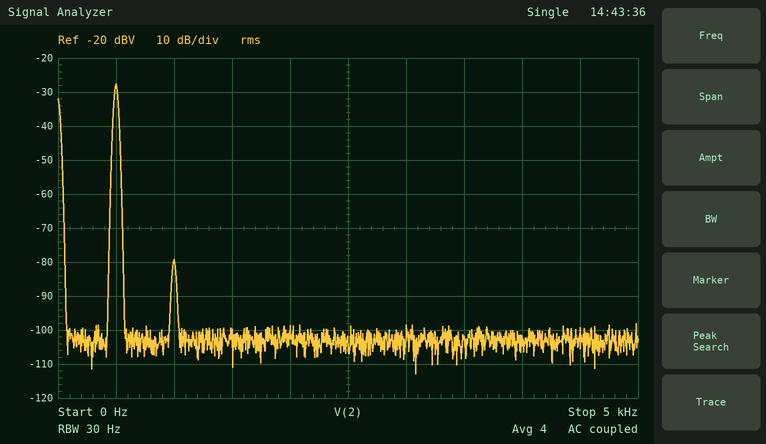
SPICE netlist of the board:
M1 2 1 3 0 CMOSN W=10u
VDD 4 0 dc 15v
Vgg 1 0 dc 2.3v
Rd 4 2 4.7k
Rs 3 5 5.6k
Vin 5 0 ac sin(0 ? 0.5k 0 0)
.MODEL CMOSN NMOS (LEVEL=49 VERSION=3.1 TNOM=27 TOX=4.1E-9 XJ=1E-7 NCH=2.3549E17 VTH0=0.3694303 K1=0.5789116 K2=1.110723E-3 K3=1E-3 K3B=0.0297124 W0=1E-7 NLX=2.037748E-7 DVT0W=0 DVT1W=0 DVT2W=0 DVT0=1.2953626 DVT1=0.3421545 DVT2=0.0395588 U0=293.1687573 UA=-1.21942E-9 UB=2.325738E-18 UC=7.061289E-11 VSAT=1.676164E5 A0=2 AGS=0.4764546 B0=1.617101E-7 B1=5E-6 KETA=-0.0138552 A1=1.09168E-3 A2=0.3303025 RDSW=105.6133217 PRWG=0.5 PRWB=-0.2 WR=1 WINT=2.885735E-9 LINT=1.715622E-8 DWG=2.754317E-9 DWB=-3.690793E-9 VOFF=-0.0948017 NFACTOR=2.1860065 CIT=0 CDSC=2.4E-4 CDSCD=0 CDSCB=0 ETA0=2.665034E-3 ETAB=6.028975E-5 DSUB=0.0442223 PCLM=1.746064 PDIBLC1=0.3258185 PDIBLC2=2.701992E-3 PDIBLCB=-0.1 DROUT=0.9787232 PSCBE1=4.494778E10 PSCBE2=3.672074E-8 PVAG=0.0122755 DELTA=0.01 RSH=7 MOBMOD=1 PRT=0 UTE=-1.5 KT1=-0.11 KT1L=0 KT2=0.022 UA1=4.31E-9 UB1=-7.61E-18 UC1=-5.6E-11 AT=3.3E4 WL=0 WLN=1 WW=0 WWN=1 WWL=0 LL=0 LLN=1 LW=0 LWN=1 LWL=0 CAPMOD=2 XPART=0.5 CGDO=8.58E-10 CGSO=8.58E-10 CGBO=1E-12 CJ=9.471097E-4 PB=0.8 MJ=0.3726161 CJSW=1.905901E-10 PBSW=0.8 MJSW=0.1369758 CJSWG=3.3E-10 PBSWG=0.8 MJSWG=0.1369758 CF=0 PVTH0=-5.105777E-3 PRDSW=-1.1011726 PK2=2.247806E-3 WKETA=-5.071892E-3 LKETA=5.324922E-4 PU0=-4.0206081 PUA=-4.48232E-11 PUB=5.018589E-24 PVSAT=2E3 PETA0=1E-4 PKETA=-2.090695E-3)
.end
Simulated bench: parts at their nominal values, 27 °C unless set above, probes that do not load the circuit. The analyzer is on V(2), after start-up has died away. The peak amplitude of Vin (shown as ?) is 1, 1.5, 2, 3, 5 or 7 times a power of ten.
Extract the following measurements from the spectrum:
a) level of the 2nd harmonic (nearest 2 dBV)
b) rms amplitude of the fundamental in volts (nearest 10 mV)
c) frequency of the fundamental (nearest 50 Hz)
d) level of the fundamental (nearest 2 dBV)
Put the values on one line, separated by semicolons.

-80 dBV; 40 mV; 500 Hz; -28 dBV
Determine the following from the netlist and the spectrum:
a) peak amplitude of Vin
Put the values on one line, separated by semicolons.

100 mV
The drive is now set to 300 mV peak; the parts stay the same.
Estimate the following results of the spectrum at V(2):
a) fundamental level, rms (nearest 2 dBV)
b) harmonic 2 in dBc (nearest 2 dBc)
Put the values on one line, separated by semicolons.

-18 dBV; -42 dBc
